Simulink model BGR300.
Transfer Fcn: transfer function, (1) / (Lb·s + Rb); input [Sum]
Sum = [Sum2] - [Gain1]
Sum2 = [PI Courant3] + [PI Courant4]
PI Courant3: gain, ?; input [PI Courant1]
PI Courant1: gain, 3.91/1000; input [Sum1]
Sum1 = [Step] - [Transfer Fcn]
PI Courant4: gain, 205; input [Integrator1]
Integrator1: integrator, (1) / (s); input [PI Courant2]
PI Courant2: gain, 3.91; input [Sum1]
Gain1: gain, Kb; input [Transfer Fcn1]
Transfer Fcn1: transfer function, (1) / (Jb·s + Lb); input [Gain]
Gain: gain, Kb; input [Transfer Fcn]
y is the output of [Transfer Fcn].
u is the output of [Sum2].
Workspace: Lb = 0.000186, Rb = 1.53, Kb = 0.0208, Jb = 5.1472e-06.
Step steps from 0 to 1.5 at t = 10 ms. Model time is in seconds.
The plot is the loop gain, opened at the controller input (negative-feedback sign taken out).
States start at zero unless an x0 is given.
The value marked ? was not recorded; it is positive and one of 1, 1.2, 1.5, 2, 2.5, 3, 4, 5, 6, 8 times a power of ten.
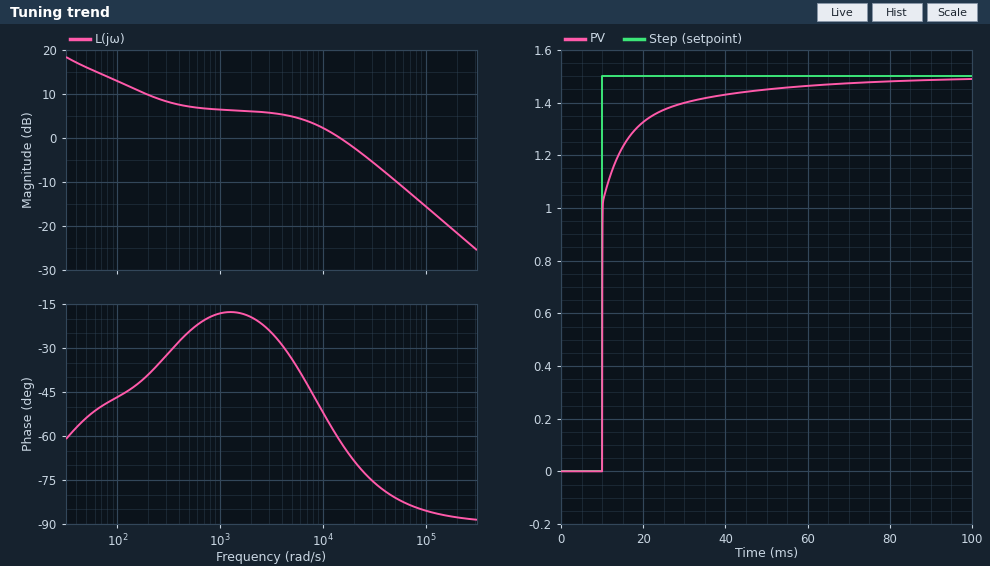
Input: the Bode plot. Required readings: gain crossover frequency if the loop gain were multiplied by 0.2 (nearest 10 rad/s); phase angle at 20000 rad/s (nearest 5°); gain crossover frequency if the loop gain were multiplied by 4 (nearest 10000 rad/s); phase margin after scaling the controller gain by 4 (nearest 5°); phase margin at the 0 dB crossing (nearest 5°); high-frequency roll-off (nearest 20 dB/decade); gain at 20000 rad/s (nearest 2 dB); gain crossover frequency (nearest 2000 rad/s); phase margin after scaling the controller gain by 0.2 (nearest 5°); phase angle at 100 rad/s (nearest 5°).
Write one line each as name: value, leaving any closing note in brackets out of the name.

gain crossover frequency if the loop gain were multiplied by 0.2: 80 rad/s
phase angle at 20000 rad/s: -70°
gain crossover frequency if the loop gain were multiplied by 4: 70000 rad/s
phase margin after scaling the controller gain by 4: 95°
phase margin at the 0 dB crossing: 120°
high-frequency roll-off: -20 dB/decade
gain at 20000 rad/s: -2 dB
gain crossover frequency: 14000 rad/s
phase margin after scaling the controller gain by 0.2: 130°
phase angle at 100 rad/s: -45°
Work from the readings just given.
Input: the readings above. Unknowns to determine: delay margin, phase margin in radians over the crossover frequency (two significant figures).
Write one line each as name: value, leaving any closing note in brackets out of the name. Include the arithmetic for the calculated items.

delay margin, phase margin in radians over the crossover frequency: 120 × π / 180 / 14000 = 0.00015 s
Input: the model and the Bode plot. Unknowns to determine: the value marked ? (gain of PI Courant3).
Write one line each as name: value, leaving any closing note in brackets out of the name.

the value marked ?: 800
